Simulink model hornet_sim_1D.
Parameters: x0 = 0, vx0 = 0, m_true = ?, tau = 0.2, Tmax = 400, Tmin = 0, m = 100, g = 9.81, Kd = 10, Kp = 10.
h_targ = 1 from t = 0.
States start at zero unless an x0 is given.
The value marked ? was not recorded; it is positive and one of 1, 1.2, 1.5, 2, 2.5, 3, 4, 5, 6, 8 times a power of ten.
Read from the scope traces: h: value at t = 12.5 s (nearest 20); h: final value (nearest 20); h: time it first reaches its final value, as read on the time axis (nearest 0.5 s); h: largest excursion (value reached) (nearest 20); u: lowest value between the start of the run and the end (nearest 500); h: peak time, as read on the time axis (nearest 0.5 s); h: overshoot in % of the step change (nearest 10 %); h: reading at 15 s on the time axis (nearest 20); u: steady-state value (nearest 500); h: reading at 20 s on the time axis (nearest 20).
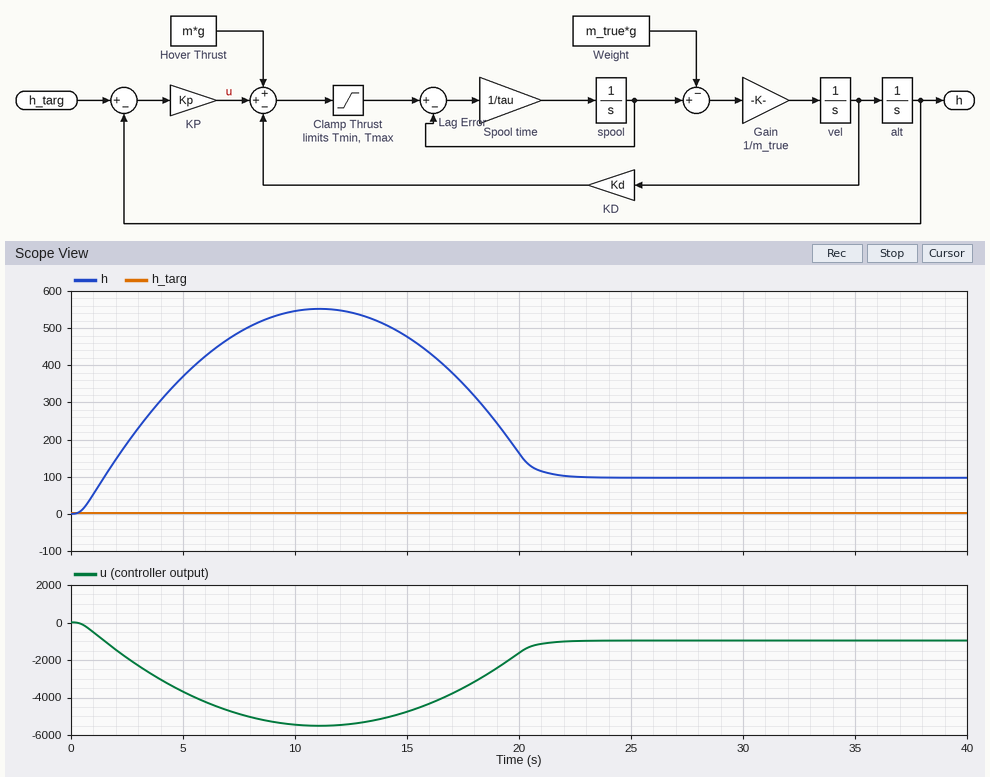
540
100
1.5 s
560
-5500
11.0 s
470 %
480
-1000
160
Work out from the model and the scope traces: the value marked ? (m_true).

2
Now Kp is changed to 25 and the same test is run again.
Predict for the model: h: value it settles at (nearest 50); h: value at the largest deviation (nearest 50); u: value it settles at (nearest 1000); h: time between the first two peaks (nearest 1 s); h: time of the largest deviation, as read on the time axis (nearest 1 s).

50
450
-1000
13 s
10 s
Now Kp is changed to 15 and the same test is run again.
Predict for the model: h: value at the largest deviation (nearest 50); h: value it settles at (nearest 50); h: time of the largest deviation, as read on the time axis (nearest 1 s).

500
50
11 s
